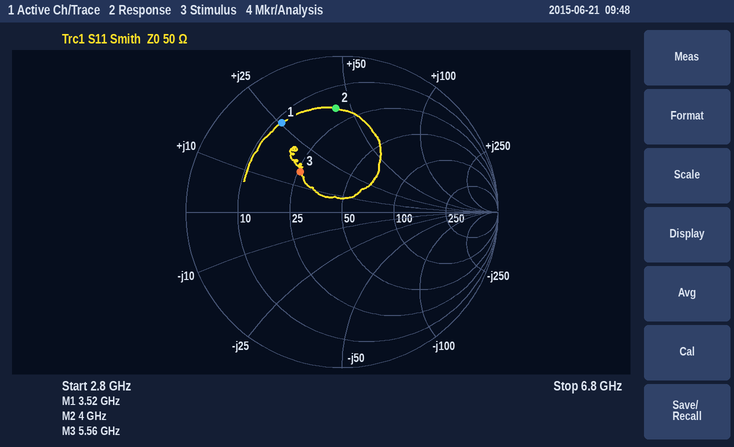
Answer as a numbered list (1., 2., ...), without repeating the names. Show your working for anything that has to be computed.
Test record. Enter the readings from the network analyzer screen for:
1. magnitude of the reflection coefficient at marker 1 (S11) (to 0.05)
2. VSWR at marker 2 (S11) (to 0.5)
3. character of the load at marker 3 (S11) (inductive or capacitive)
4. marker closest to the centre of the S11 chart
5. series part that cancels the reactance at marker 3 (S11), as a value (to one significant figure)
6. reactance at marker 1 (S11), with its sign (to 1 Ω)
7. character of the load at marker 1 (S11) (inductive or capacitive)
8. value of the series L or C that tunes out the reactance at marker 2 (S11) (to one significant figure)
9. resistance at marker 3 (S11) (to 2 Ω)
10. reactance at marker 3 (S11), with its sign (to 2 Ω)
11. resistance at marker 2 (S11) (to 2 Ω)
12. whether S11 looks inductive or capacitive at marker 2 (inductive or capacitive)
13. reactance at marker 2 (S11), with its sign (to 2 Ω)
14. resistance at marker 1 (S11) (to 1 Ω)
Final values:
1. 0.70
2. 5.0
3. inductive
4. marker 3
5. C = 1/(2π × 5.56 GHz × 16 Ω) ≈ 2 pF
6. +25 Ω
7. inductive
8. C = 1/(2π × 4 GHz × 44 Ω) ≈ 904 fF, so 900 fF to one significant figure
9. 26 Ω
10. +16 Ω
11. 18 Ω
12. inductive
13. +44 Ω
14. 12 Ω
